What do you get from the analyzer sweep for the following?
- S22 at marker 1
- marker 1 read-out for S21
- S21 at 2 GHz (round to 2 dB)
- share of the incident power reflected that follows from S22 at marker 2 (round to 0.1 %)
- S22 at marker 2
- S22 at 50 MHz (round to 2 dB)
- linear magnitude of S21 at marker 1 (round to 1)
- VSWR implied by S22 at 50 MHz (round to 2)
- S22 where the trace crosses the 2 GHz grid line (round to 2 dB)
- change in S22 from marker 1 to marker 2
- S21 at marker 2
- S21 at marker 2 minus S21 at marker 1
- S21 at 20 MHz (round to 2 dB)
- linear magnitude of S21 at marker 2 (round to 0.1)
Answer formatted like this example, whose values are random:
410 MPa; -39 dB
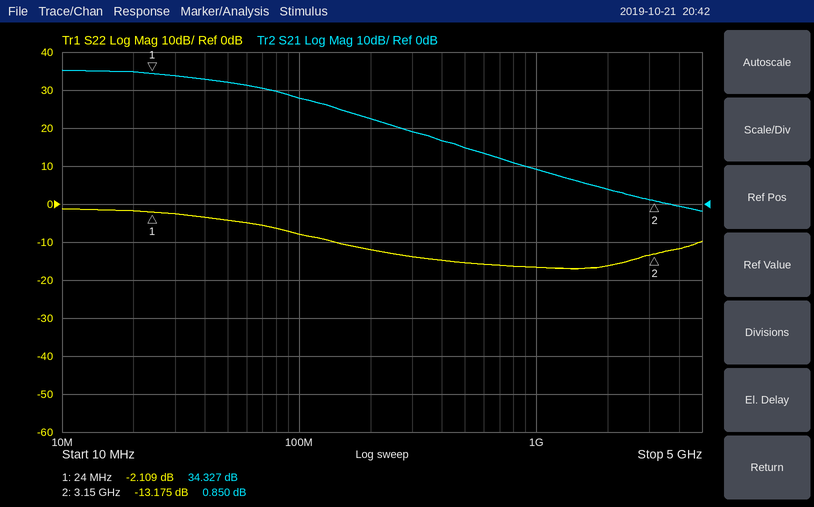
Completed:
-2.109 dB; 34.327 dB; 4 dB; 4.8 %; -13.175 dB; -4 dB; 52; 4; -16 dB; -11.066 dB; 0.850 dB; -33.477 dB; 34 dB; 1.1
